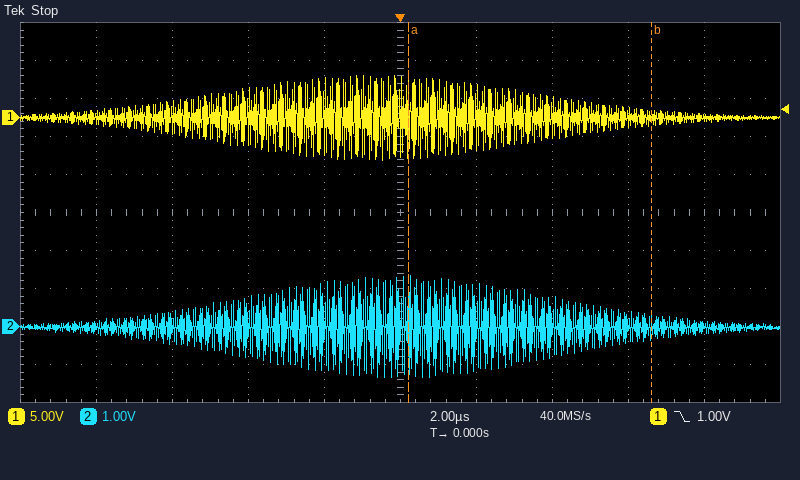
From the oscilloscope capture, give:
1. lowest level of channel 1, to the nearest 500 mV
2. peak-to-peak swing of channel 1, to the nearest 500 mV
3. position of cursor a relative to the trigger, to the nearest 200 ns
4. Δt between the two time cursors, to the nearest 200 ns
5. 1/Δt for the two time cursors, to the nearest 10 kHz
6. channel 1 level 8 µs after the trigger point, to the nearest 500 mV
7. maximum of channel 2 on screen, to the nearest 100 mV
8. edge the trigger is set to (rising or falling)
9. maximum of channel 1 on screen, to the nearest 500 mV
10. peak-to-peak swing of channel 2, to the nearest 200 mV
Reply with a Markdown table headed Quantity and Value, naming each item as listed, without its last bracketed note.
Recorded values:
| Quantity | Value |
|---|---|
| lowest level of channel 1, to the nearest 500 mV | -5.5 V |
| peak-to-peak swing of channel 1, to the nearest 500 mV | 11.0 V |
| position of cursor a relative to the trigger, to the nearest 200 ns | +200 ns |
| Δt between the two time cursors, to the nearest 200 ns | 6.4 µs |
| 1/Δt for the two time cursors, to the nearest 10 kHz | 160 kHz |
| channel 1 level 8 µs after the trigger point, to the nearest 500 mV | 0.0 V |
| maximum of channel 2 on screen, to the nearest 100 mV | 1.3 V |
| edge the trigger is set to | falling |
| maximum of channel 1 on screen, to the nearest 500 mV | 5.5 V |
| peak-to-peak swing of channel 2, to the nearest 200 mV | 2.6 V |
